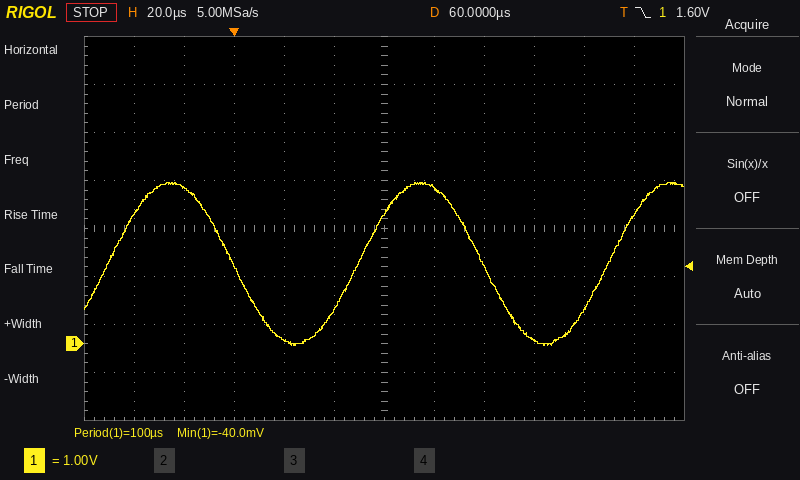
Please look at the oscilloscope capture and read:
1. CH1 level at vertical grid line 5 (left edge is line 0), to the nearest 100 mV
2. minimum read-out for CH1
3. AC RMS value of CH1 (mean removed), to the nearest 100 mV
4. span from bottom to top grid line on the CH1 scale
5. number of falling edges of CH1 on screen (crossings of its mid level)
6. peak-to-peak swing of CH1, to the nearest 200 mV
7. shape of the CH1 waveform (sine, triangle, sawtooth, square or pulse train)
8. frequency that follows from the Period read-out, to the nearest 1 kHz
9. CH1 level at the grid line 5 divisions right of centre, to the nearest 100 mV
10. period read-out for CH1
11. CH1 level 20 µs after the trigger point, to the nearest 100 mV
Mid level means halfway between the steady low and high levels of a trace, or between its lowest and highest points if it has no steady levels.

700 mV
-40.0 mV
1.2 V
8 V
2
3.4 V
sine
10 kHz
2.7 V
100 µs
100 mV
